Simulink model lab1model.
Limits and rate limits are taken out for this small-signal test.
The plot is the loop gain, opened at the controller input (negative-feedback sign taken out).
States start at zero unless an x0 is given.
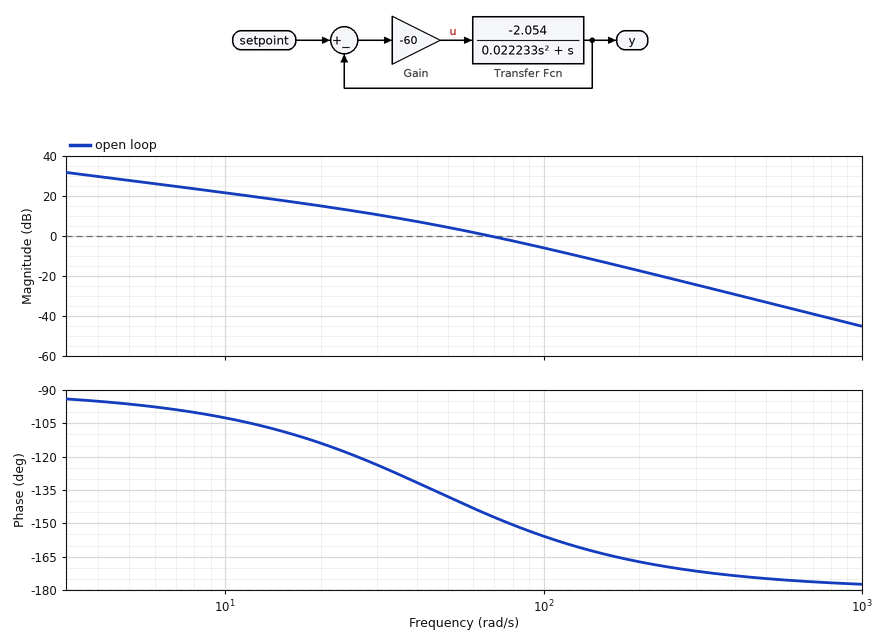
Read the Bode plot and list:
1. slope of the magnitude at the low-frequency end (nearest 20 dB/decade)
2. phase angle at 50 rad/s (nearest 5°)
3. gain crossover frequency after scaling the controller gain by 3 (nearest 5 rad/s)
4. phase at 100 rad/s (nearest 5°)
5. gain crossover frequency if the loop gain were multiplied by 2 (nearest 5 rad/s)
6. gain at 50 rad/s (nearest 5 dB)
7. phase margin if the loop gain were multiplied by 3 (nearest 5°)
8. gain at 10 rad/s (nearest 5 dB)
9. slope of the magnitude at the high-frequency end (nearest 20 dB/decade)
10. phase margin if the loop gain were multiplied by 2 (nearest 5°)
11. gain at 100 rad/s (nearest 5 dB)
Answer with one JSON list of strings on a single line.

["-20 dB/decade", "-140°", "125 rad/s", "-155°", "100 rad/s", "5 dB", "20°", "20 dB", "-40 dB/decade", "25°", "-5 dB"]
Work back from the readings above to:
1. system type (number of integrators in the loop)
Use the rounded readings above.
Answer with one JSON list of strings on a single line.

["1"]
